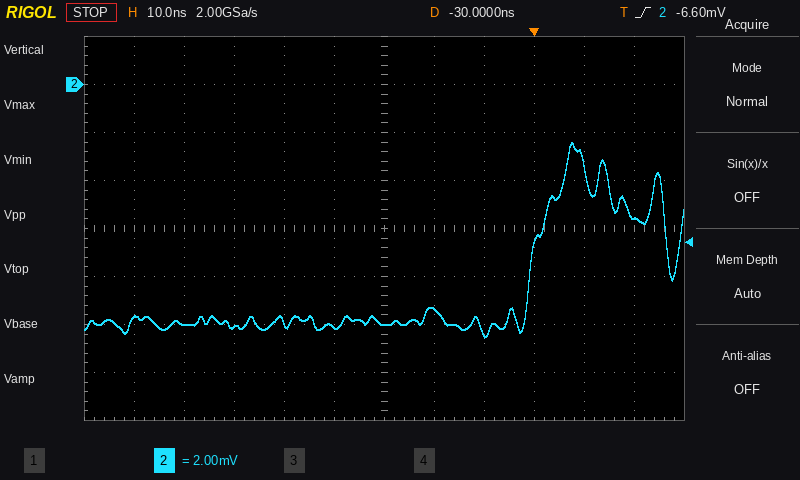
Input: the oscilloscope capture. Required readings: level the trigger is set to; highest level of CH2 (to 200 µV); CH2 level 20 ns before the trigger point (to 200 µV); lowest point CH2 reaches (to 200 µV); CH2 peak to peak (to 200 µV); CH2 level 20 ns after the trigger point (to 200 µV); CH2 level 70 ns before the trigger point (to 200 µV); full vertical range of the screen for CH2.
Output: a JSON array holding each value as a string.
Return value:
["-6.60 mV", "-2.4 mV", "-9.4 mV", "-10.6 mV", "8.2 mV", "-5.6 mV", "-10.0 mV", "16 mV"]
